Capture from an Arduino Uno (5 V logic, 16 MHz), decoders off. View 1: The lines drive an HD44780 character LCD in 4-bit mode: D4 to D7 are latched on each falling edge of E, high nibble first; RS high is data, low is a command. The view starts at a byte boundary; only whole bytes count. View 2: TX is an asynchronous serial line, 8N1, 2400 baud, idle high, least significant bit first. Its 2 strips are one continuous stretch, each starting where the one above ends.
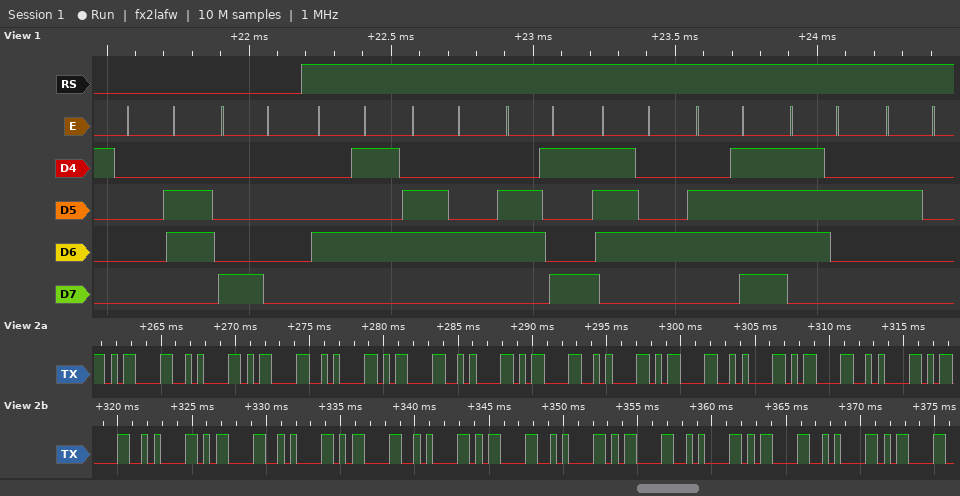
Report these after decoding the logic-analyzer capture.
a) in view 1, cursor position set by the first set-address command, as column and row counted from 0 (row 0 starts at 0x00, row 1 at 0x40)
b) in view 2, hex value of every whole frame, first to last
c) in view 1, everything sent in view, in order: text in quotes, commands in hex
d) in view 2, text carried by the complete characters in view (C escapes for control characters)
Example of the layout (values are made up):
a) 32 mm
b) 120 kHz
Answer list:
a) column 0, row 0
b) 0D 0A 0D 0A 0D 0A 0D 0A 0D 0A 0D 0A 0D 0A 0D 0A 0D 0A 0D 0A 0D 0A 0D 0A 0D
c) 0x06 0x80 "Editor "
d) "\r\n\r\n\r\n\r\n\r\n\r\n\r\n\r\n\r\n\r\n\r\n\r\n\r"
